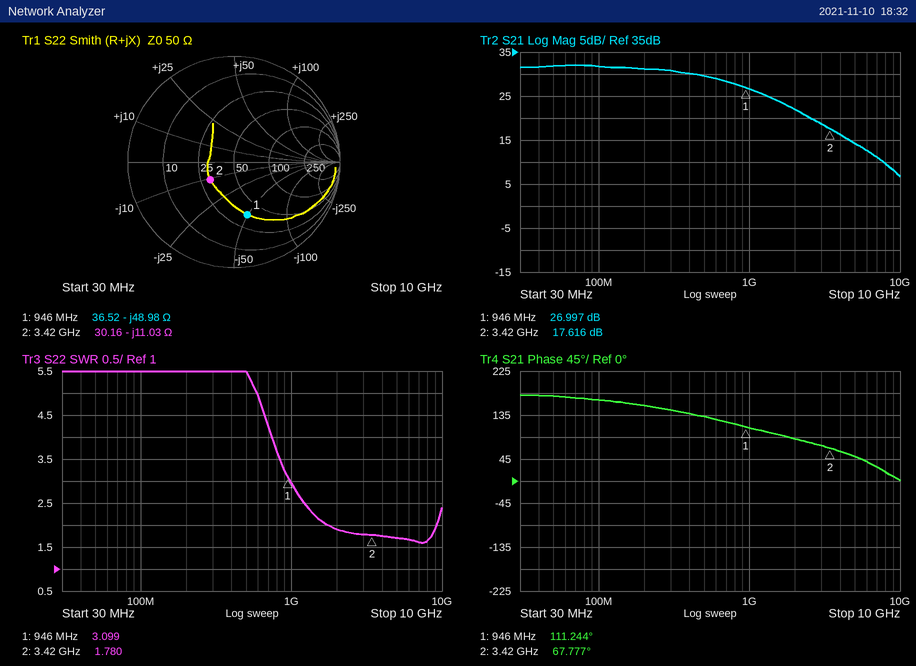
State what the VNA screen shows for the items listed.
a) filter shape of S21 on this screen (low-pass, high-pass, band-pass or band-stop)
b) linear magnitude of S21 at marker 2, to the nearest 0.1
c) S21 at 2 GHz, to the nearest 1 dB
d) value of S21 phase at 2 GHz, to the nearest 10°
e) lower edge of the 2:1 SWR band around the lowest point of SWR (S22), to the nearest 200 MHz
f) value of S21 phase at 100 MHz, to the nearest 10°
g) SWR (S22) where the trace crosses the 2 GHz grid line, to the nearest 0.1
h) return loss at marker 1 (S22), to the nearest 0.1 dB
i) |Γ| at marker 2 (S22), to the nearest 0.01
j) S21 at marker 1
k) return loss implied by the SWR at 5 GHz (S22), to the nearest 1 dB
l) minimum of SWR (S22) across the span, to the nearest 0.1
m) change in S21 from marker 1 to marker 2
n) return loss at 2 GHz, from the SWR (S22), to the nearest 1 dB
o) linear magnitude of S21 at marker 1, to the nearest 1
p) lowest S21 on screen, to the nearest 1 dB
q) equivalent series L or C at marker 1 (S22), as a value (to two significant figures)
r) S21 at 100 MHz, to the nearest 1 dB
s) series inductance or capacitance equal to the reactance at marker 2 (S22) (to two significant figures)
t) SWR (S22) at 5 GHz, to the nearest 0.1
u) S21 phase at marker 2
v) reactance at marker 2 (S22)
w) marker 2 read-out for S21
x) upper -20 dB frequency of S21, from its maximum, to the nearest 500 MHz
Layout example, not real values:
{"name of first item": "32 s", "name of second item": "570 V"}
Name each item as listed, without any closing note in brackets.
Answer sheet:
{"filter shape of S21 on this screen": "low-pass", "linear magnitude of S21 at marker 2, to the nearest 0.1": "7.6", "S21 at 2 GHz, to the nearest 1 dB": "22 dB", "value of S21 phase at 2 GHz, to the nearest 10°": "90°", "lower edge of the 2:1 SWR band around the lowest point of SWR (S22), to the nearest 200 MHz": "1.8 GHz", "value of S21 phase at 100 MHz, to the nearest 10°": "170°", "SWR (S22) where the trace crosses the 2 GHz grid line, to the nearest 0.1": "1.9", "return loss at marker 1 (S22), to the nearest 0.1 dB": "5.8 dB", "|Γ| at marker 2 (S22), to the nearest 0.01": "0.28", "S21 at marker 1": "26.997 dB", "return loss implied by the SWR at 5 GHz (S22), to the nearest 1 dB": "12 dB", "minimum of SWR (S22) across the span, to the nearest 0.1": "1.6", "change in S21 from marker 1 to marker 2": "-9.381 dB", "return loss at 2 GHz, from the SWR (S22), to the nearest 1 dB": "10 dB", "linear magnitude of S21 at marker 1, to the nearest 1": "22", "lowest S21 on screen, to the nearest 1 dB": "7 dB", "equivalent series L or C at marker 1 (S22), as a value": "3.4 pF", "S21 at 100 MHz, to the nearest 1 dB": "32 dB", "series inductance or capacitance equal to the reactance at marker 2 (S22)": "4.2 pF", "SWR (S22) at 5 GHz, to the nearest 0.1": "1.7", "S21 phase at marker 2": "67.777°", "reactance at marker 2": "-11.03 Ω", "marker 2 read-out for S21": "17.616 dB", "upper -20 dB frequency of S21, from its maximum, to the nearest 500 MHz": "6.5 GHz"}
